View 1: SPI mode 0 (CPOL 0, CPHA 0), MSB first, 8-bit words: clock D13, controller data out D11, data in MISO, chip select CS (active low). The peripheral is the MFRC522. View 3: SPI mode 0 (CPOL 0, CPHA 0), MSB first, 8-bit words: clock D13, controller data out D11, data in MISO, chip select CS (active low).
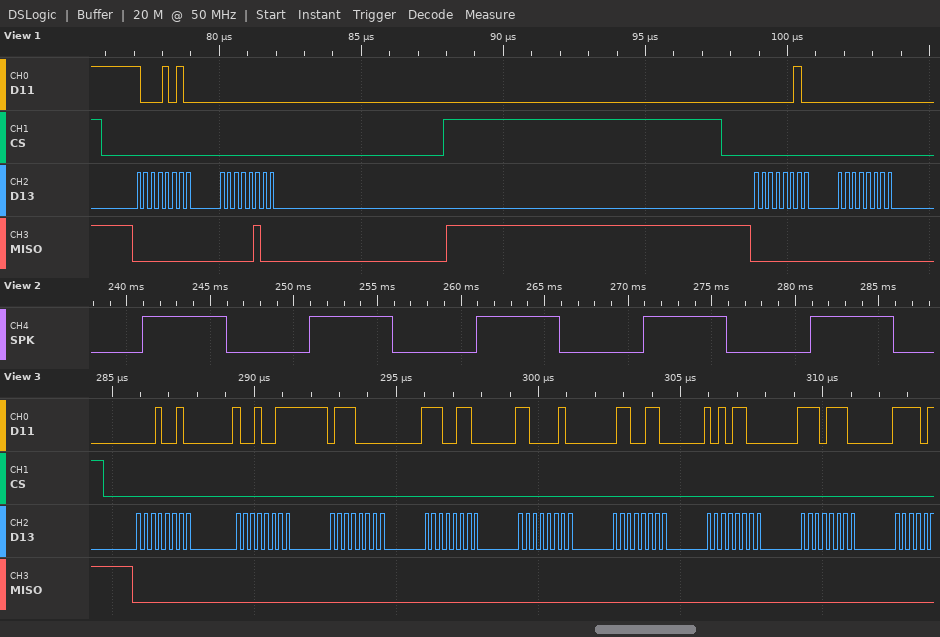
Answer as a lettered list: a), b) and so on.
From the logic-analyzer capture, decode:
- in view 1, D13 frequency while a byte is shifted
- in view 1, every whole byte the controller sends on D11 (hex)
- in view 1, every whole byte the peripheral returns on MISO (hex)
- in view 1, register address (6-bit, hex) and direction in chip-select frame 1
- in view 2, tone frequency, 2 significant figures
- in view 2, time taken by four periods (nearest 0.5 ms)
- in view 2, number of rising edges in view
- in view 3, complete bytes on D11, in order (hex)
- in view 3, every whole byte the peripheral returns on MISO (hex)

a) 4 MHz
b) 0x8A 0x00 0x02 0x00
c) 0x00 0x04 0x00 0x00
d) 0x05 read
e) 100 Hz
f) 40.0 ms
g) 5
h) 12 93 70 E6 C2 66 AC EE
i) 00 00 00 00 00 00 00 00
